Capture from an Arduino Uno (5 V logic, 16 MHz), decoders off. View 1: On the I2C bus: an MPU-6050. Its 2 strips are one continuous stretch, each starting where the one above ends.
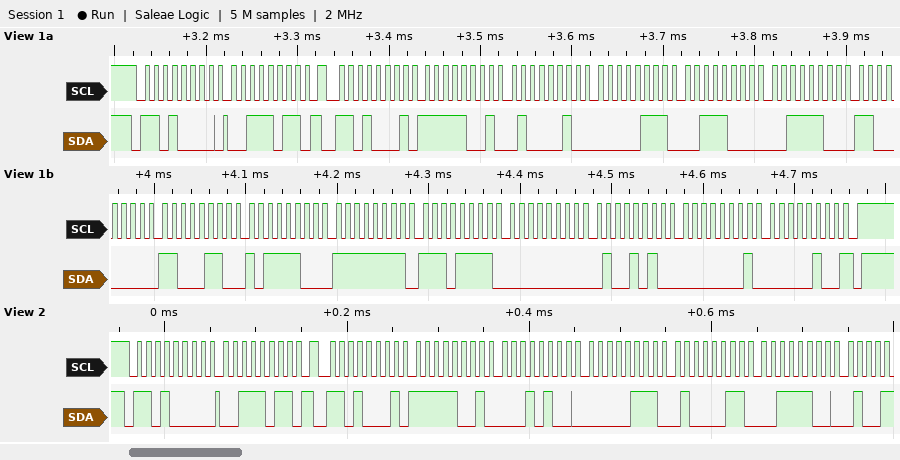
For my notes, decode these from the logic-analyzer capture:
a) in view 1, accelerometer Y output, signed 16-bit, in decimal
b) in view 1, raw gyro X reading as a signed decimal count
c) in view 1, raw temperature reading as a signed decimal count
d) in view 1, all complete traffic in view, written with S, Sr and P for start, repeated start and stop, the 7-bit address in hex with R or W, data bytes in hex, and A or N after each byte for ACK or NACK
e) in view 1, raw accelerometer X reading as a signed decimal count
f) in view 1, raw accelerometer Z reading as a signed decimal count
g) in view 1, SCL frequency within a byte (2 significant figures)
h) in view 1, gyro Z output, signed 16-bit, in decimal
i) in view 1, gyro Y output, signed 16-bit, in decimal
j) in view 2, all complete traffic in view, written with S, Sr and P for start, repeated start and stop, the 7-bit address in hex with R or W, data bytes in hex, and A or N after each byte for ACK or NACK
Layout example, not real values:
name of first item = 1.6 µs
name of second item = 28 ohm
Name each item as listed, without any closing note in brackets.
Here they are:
in view 1, accelerometer Y output, signed 16-bit, in decimal = 1848
in view 1, raw gyro X reading as a signed decimal count = -17
in view 1, raw temperature reading as a signed decimal count = -14660
in view 1, all complete traffic in view, written with S, Sr and P for start, repeated start and stop, the 7-bit address in hex with R or W, data bytes in hex, and A or N after each byte for ACK or NACK = S 68W A 3B A Sr 68R A F9 A 42 A 07 A 38 A 3C A C0 A C6 A BC A FF A EF A 00 A 4A A 01 A 04 N P
in view 1, raw accelerometer X reading as a signed decimal count = -1726
in view 1, raw accelerometer Z reading as a signed decimal count = 15552
in view 1, SCL frequency within a byte = 100 kHz
in view 1, gyro Z output, signed 16-bit, in decimal = 260
in view 1, gyro Y output, signed 16-bit, in decimal = 74
in view 2, all complete traffic in view, written with S, Sr and P for start, repeated start and stop, the 7-bit address in hex with R or W, data bytes in hex, and A or N after each byte for ACK or NACK = S 68W A 3B A Sr 68R A F9 A 14 A 07 A 43 A 3C A
